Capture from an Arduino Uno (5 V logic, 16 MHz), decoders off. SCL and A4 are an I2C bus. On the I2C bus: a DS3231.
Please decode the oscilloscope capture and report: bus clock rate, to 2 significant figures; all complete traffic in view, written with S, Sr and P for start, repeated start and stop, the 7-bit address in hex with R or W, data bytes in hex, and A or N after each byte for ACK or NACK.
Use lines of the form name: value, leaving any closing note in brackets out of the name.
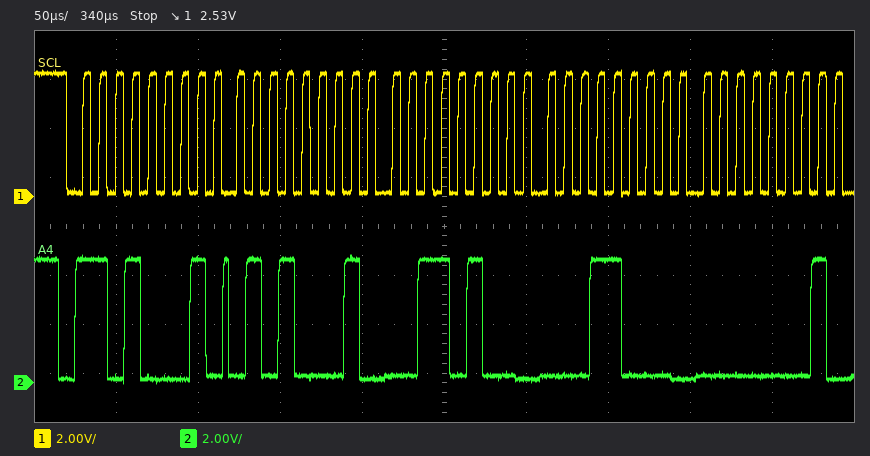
bus clock rate, to 2 significant figures: 100 kHz
all complete traffic in view, written with S, Sr and P for start, repeated start and stop, the 7-bit address in hex with R or W, data bytes in hex, and A or N after each byte for ACK or NACK: S 68R A 51 A 34 A 18 A 01 A
